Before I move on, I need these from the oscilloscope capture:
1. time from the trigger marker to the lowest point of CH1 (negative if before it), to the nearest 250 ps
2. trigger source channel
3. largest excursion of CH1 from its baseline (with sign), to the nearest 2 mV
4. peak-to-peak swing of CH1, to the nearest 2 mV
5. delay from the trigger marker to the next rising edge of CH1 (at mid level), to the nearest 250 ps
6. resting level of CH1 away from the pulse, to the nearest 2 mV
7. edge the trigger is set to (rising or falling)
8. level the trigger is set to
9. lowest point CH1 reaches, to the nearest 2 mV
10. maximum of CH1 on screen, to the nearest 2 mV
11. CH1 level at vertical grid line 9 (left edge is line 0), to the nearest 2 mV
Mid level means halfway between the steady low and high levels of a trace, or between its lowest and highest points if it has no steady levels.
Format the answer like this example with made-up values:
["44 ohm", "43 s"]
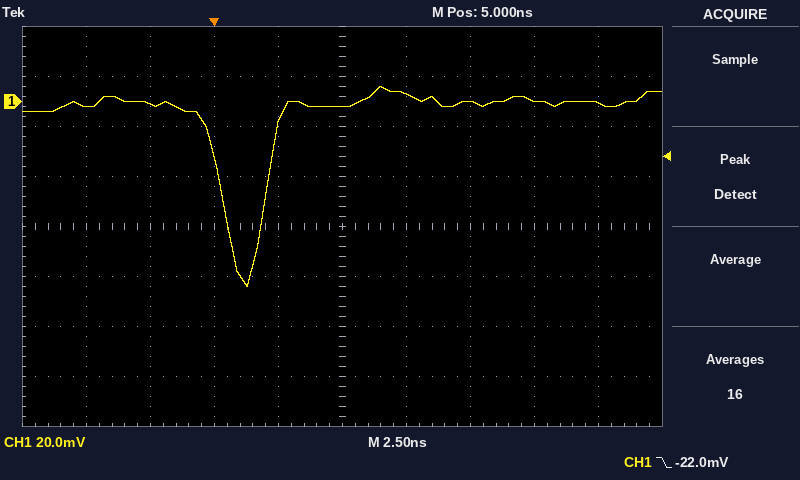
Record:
["+1.25 ns", "CH1", "-74 mV", "80 mV", "2.00 ns", "0 mV", "falling", "-22.0 mV", "-74 mV", "6 mV", "0 mV"]
